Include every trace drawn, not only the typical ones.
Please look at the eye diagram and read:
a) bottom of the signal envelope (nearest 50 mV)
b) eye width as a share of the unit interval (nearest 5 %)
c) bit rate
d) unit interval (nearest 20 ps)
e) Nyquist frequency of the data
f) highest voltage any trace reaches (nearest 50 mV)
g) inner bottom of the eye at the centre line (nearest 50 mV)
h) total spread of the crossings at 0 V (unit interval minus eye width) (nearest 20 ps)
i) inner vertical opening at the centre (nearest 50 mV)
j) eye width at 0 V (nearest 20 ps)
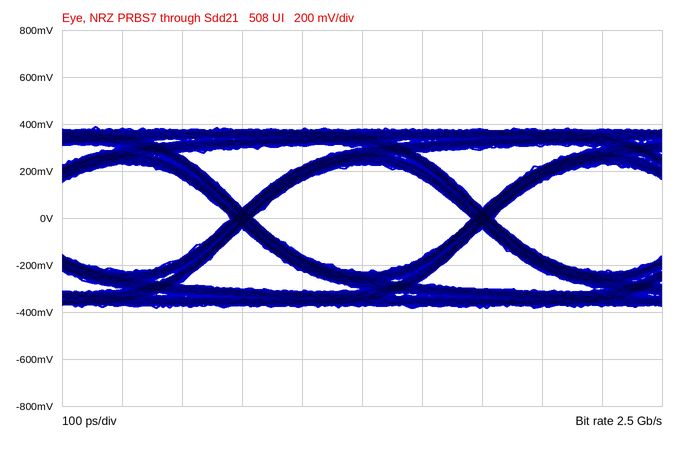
-400 mV
90 %
2.5 Gb/s
400 ps
1.25 GHz
400 mV
-250 mV
40 ps
450 mV
360 ps
